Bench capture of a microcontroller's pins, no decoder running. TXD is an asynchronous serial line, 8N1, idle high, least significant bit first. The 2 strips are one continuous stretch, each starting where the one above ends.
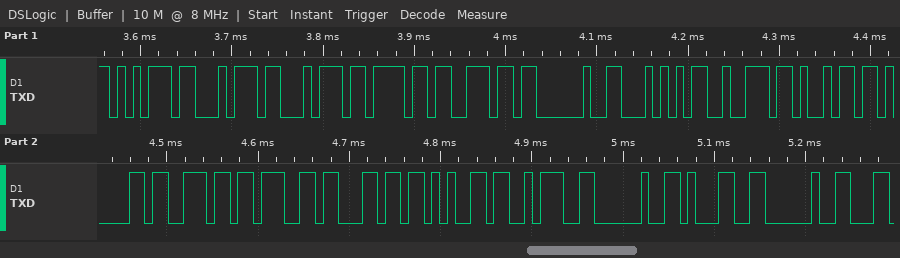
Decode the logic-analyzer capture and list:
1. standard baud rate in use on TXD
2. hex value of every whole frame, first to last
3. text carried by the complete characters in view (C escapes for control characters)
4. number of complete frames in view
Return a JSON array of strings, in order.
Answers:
["115200 baud", "75 74 74 6F 6E 20 54 72 69 61 6E 67 6C 65 3A 20 31 20", "\"utton Triangle: 1 \"", "18"]
